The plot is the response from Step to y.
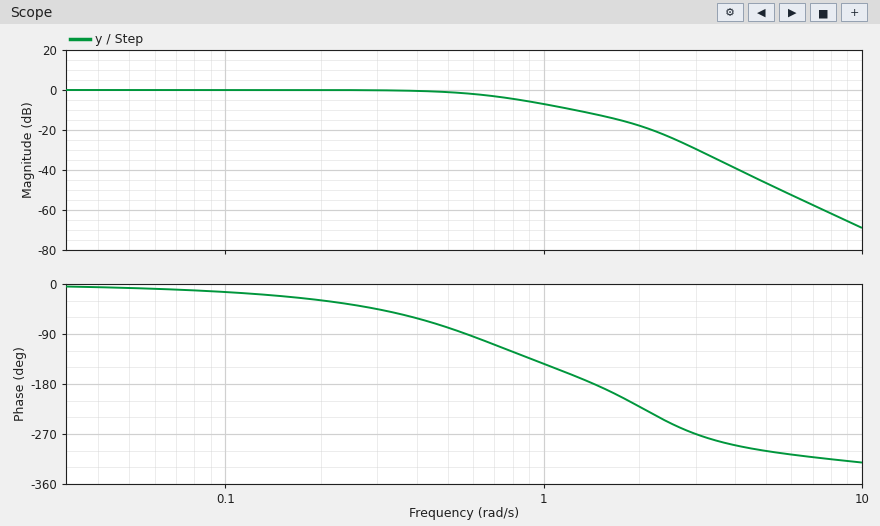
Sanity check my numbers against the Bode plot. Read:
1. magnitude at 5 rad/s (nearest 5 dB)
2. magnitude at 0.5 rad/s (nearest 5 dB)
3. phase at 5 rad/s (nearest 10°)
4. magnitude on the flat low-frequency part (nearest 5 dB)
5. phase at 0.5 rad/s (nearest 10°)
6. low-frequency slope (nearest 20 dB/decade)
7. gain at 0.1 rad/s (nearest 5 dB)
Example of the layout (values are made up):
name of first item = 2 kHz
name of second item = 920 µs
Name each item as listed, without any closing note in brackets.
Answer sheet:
magnitude at 5 rad/s = -45 dB
magnitude at 0.5 rad/s = 0 dB
phase at 5 rad/s = -300°
magnitude on the flat low-frequency part = 0 dB
phase at 0.5 rad/s = -80°
low-frequency slope = 0 dB/decade
gain at 0.1 rad/s = 0 dB
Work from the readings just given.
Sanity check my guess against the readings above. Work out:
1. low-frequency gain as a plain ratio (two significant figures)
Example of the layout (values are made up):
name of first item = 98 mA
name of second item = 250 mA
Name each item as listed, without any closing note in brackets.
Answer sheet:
low-frequency gain as a plain ratio = 1.0
